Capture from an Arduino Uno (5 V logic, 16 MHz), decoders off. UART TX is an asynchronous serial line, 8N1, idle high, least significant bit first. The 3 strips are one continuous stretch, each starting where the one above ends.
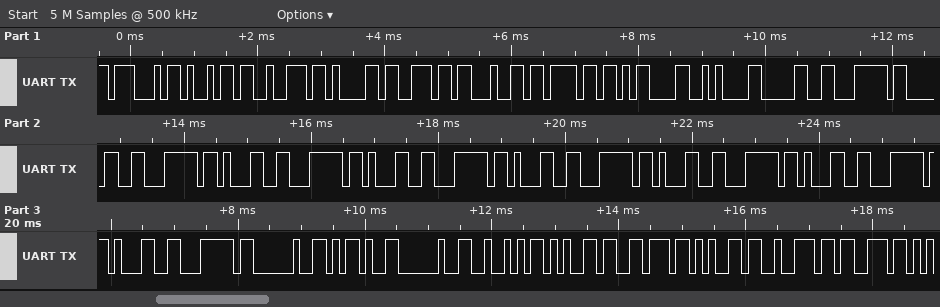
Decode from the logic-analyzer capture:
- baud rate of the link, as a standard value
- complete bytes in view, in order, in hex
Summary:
9600 baud
47 69 72 61 6E 64 6F 0D 0A 30 7C 30 7C 31 7C 31 7C 31 7C 31 7C 31 7C 31 7C 20 2D 20 52 65 76 65 72 73
